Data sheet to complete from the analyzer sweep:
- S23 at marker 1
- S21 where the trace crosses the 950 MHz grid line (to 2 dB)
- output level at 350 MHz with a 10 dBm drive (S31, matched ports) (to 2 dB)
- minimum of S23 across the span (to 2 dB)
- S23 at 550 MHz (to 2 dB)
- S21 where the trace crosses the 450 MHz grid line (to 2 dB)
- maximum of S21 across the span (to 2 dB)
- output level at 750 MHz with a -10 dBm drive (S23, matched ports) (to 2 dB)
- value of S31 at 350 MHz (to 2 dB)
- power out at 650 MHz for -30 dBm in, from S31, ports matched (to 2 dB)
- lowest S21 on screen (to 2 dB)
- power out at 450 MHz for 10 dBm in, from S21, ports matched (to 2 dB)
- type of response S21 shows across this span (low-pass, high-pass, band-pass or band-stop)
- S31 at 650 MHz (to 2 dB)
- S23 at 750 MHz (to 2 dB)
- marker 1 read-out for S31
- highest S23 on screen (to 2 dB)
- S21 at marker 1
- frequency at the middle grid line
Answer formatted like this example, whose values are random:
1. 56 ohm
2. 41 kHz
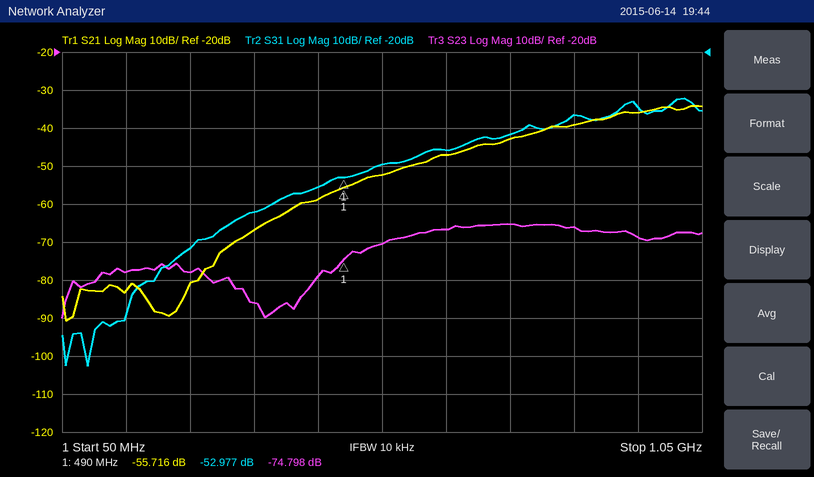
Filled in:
1. -74.798 dB
2. -36 dB
3. -52 dBm
4. -90 dB
5. -70 dB
6. -58 dB
7. -34 dB
8. -76 dBm
9. -62 dB
10. -76 dBm
11. -90 dB
12. -48 dBm
13. high-pass
14. -46 dB
15. -66 dB
16. -52.977 dB
17. -66 dB
18. -55.716 dB
19. 550 MHz
